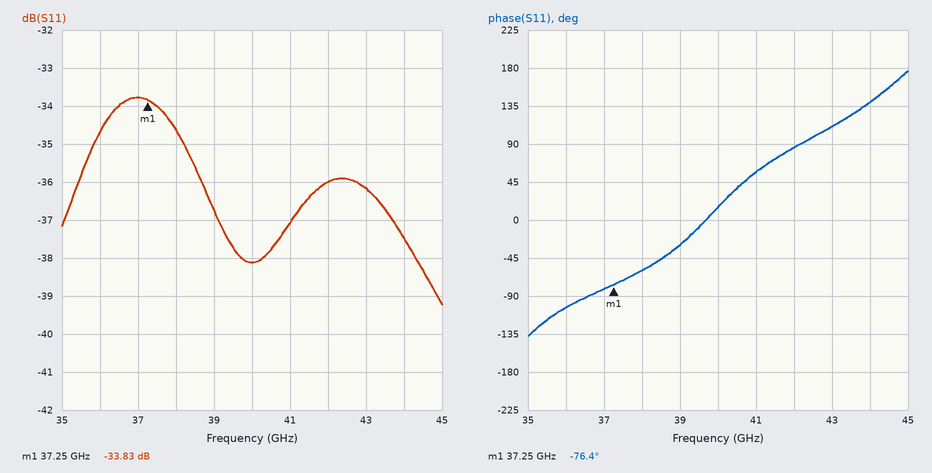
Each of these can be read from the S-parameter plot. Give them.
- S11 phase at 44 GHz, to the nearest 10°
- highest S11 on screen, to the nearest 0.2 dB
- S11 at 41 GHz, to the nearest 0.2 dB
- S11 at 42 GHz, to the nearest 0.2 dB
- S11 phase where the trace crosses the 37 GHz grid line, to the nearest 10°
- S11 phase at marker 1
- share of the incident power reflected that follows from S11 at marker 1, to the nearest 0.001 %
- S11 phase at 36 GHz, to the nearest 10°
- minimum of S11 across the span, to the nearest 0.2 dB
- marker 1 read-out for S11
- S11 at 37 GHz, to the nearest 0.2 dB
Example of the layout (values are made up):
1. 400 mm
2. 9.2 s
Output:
1. 140°
2. -33.8 dB
3. -37.0 dB
4. -36.0 dB
5. -80°
6. -76.4°
7. 0.041 %
8. -100°
9. -39.2 dB
10. -33.83 dB
11. -33.8 dB
